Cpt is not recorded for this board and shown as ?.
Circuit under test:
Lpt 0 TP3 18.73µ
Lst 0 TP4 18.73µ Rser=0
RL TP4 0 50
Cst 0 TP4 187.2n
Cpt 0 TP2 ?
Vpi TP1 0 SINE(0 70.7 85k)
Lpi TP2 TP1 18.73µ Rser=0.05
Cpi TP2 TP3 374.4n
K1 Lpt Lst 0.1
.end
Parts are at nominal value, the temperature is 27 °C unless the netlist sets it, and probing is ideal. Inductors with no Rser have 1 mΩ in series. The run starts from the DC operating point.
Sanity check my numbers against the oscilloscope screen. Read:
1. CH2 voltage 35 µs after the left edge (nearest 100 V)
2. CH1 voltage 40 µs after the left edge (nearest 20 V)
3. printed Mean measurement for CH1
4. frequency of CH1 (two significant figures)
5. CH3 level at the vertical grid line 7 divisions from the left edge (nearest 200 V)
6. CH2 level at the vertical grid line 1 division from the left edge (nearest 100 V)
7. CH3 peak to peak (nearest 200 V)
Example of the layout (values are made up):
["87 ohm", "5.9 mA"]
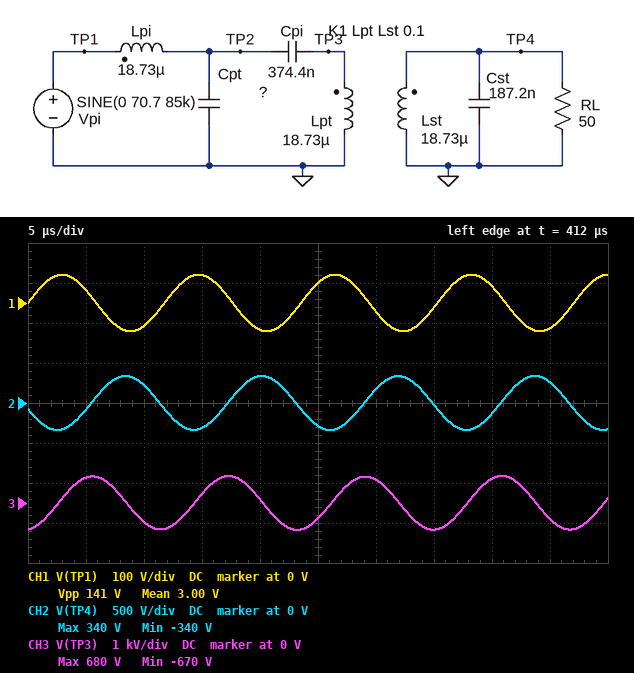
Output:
["0 V", "40 V", "3.00 V", "85 kHz", "-600 V", "-100 V", "1.4 kV"]
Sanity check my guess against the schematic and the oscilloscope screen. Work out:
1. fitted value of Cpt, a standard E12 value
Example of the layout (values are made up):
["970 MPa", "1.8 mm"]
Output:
["560 nF"]
